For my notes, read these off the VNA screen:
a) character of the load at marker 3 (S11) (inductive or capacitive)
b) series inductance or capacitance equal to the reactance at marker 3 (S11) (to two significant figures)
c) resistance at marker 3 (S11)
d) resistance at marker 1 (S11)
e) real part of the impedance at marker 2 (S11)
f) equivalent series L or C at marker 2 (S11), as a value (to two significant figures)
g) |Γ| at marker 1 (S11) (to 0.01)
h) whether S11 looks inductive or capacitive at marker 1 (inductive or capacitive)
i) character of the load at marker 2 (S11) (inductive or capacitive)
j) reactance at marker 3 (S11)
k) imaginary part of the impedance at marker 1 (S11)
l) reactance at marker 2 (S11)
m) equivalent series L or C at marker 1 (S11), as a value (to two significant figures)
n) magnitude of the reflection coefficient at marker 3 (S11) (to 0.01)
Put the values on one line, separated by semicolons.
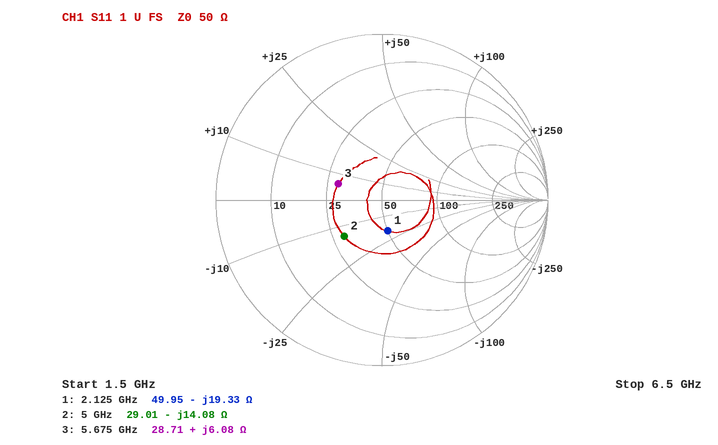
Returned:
inductive; 170 pH; 28.71 Ω; 49.95 Ω; 29.01 Ω; 2.3 pF; 0.19; capacitive; capacitive; +6.08 Ω; -19.33 Ω; -14.08 Ω; 3.9 pF; 0.28
